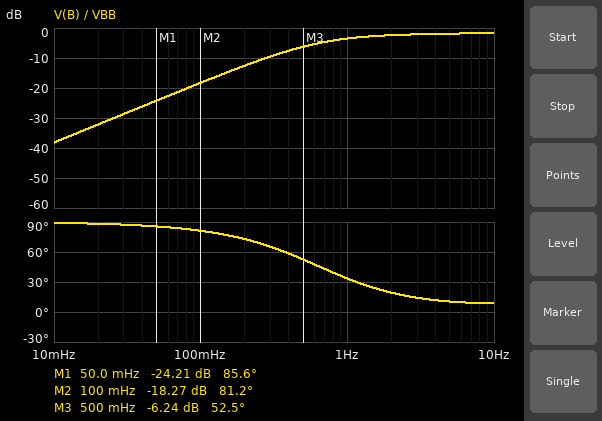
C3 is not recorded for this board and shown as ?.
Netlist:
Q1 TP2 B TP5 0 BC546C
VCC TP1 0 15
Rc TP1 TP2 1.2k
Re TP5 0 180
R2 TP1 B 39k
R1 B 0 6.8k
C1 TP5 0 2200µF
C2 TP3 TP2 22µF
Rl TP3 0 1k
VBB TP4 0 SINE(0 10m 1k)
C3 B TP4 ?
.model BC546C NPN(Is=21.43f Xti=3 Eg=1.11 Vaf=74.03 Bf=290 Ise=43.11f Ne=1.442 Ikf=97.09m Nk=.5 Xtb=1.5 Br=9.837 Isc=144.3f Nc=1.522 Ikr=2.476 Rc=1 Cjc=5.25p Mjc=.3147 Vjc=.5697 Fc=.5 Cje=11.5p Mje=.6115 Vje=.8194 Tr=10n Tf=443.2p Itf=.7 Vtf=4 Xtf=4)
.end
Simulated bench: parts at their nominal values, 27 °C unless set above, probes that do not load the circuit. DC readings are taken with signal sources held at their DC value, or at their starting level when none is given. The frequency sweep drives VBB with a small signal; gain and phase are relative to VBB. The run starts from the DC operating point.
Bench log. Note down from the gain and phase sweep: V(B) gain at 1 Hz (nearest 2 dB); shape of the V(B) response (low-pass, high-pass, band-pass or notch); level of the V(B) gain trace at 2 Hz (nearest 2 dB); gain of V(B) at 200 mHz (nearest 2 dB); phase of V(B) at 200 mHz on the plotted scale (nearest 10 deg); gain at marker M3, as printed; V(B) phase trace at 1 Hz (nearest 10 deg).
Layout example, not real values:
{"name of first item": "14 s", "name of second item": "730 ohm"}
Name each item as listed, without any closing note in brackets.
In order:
{"V(B) gain at 1 Hz": "-4 dB", "shape of the V(B) response": "high-pass", "level of the V(B) gain trace at 2 Hz": "-2 dB", "gain of V(B) at 200 mHz": "-12 dB", "phase of V(B) at 200 mHz on the plotted scale": "70 deg", "gain at marker M3, as printed": "-6.24 dB", "V(B) phase trace at 1 Hz": "30 deg"}
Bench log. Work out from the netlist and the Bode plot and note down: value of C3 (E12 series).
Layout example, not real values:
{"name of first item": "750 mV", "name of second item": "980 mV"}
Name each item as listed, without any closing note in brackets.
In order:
{"value of C3": "39 µF"}
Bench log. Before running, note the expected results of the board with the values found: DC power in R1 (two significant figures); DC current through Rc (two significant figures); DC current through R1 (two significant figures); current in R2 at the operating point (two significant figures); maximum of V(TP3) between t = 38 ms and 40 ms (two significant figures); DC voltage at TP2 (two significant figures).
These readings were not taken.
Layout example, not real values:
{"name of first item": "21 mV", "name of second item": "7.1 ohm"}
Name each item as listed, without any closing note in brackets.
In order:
{"DC power in R1": "620 µW", "DC current through Rc": "7.5 mA", "DC current through R1": "300 µA", "current in R2 at the operating point": "330 µA", "maximum of V(TP3) between t = 38 ms and 40 ms": "1.3 V", "DC voltage at TP2": "6.0 V"}
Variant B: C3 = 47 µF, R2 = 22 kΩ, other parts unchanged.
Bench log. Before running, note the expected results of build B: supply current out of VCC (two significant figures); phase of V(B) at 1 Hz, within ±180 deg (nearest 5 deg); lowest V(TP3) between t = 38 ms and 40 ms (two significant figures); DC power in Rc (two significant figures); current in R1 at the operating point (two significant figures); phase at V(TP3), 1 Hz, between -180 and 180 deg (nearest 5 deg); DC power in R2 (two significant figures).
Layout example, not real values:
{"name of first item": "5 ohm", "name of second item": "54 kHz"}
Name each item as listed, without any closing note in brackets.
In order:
{"supply current out of VCC": "11 mA", "phase of V(B) at 1 Hz, within ±180 deg": "40 deg", "lowest V(TP3) between t = 38 ms and 40 ms": "-540 mV", "DC power in Rc": "140 mW", "current in R1 at the operating point": "390 µA", "phase at V(TP3), 1 Hz, between -180 and 180 deg": "15 deg", "DC power in R2": "6.9 mW"}
